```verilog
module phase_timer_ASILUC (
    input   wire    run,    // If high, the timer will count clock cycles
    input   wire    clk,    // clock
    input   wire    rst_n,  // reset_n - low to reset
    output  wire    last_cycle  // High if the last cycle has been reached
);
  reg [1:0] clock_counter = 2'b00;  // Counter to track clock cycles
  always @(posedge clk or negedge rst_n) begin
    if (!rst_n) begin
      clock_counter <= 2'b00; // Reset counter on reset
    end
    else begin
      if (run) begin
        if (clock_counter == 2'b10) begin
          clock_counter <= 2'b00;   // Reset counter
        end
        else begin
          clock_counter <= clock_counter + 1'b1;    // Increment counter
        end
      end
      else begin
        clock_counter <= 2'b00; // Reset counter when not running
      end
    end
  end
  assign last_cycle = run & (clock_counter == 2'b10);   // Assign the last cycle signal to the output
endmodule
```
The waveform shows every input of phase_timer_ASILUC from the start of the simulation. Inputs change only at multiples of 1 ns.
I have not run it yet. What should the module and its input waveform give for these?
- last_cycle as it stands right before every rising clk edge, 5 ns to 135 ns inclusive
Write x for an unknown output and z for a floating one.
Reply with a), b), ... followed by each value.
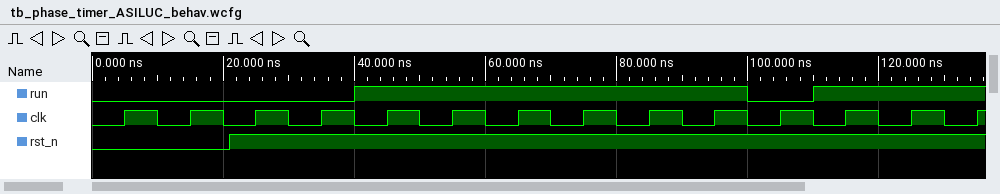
a) 0 0 0 0 0 0 1 0 0 1 0 0 0 1
